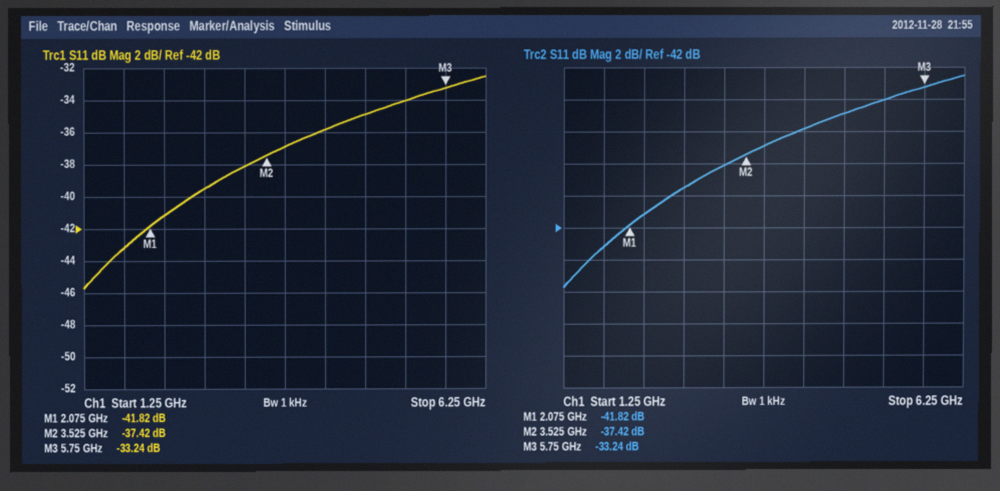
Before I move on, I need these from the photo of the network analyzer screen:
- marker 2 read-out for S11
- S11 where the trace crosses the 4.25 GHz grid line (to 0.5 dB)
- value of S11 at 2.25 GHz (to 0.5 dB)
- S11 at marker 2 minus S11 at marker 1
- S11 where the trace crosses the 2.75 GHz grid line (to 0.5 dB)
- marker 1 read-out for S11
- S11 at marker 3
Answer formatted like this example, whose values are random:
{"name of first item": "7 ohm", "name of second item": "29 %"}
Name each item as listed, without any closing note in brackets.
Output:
{"marker 2 read-out for S11": "-37.42 dB", "S11 where the trace crosses the 4.25 GHz grid line": "-36.0 dB", "value of S11 at 2.25 GHz": "-41.0 dB", "S11 at marker 2 minus S11 at marker 1": "4.40 dB", "S11 where the trace crosses the 2.75 GHz grid line": "-39.5 dB", "marker 1 read-out for S11": "-41.82 dB", "S11 at marker 3": "-33.24 dB"}
